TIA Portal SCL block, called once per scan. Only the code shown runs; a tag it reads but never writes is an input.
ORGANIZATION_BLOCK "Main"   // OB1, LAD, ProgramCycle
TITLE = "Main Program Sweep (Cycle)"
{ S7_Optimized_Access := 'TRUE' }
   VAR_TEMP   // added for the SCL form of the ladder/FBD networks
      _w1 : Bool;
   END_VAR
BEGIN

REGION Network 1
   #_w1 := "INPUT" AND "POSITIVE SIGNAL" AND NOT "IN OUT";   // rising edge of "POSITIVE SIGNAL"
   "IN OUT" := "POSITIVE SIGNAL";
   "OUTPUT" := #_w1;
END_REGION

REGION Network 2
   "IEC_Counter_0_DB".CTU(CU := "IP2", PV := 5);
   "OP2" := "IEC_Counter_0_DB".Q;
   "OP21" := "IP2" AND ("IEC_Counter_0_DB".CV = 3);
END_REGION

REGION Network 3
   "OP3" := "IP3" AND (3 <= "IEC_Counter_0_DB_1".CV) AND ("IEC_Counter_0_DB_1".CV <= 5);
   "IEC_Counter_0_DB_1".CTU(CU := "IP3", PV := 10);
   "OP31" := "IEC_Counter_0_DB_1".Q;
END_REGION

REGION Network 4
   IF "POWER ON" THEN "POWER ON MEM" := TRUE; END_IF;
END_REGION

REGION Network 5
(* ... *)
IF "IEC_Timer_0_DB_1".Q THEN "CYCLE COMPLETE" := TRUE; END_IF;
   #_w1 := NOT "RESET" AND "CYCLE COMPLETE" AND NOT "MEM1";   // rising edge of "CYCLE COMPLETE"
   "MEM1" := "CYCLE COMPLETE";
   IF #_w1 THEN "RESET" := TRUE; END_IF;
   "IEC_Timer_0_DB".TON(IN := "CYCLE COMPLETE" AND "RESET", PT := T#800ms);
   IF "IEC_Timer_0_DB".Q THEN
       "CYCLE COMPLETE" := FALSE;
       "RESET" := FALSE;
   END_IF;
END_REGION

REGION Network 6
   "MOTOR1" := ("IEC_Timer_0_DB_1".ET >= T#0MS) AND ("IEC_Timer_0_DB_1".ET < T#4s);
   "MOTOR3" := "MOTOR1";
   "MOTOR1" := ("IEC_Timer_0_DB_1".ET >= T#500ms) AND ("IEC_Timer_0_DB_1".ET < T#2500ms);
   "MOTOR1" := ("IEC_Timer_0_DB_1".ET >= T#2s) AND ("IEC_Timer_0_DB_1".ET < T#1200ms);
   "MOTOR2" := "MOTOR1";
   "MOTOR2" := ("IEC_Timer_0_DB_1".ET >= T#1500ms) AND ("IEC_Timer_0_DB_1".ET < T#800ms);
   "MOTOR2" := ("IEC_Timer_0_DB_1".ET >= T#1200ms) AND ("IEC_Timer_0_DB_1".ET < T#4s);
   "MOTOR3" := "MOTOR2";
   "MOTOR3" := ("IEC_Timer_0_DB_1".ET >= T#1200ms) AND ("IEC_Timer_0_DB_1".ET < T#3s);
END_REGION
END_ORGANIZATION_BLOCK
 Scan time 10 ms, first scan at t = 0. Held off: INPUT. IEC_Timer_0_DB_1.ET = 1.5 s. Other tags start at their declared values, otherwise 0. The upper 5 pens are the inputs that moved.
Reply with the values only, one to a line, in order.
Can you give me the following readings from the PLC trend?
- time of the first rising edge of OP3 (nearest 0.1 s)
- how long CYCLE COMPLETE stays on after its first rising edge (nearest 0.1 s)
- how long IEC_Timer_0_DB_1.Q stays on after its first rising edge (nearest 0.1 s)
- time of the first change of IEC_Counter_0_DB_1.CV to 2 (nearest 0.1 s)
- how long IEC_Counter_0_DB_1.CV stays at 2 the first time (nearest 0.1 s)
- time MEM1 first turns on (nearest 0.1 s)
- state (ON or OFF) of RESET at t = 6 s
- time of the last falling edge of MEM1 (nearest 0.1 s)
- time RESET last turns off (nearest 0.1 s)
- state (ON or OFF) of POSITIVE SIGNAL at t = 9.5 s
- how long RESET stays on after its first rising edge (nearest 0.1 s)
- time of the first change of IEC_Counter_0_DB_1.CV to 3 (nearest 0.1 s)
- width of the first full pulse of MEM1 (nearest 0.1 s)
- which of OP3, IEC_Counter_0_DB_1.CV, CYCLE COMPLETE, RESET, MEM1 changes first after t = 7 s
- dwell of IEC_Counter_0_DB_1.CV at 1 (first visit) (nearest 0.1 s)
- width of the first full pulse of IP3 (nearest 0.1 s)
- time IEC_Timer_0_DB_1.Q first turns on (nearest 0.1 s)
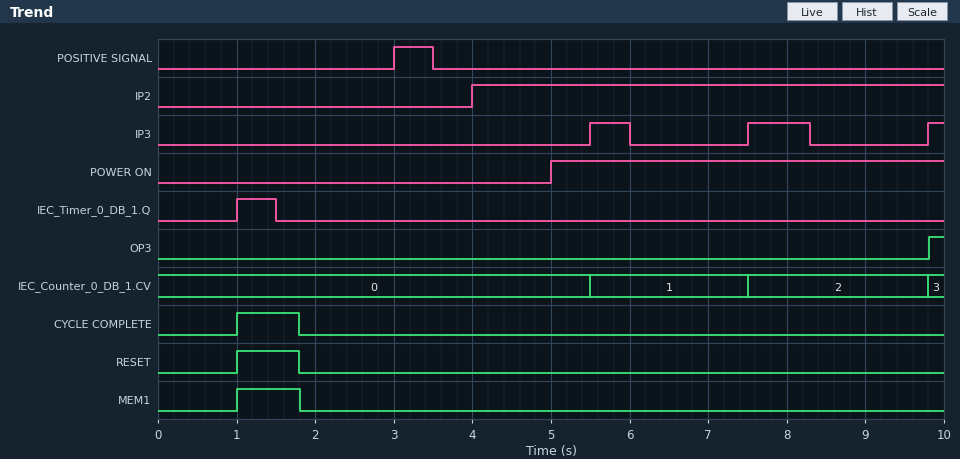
9.8 s
0.8 s
0.5 s
7.5 s
2.3 s
1.0 s
OFF
1.8 s
1.8 s
OFF
0.8 s
9.8 s
0.8 s
IEC_Counter_0_DB_1.CV
2.0 s
0.5 s
1.0 s
